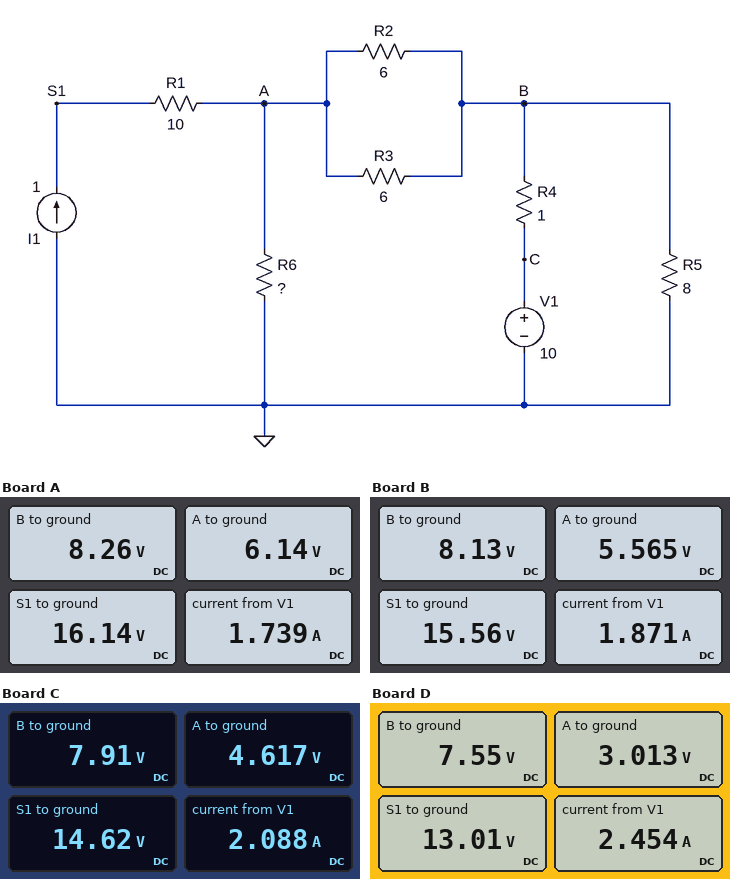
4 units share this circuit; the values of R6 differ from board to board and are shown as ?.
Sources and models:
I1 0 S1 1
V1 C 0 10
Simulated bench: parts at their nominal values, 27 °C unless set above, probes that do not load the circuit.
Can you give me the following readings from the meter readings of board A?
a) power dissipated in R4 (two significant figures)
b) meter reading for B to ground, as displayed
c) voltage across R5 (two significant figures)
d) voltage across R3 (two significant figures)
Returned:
3.0 W
8.26 V
8.3 V
2.1 V
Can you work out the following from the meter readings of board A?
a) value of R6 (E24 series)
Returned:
3.6 Ω
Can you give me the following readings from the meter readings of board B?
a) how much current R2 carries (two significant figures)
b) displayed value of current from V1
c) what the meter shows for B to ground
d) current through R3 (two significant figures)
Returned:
430 mA
1.871 A
8.13 V
430 mA
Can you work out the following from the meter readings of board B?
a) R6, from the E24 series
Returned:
3 Ω
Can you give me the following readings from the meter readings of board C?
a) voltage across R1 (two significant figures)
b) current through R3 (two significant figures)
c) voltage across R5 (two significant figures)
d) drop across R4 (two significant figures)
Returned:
10 V
550 mA
7.9 V
2.1 V
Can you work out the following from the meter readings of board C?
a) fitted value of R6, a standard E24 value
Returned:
2.2 Ω
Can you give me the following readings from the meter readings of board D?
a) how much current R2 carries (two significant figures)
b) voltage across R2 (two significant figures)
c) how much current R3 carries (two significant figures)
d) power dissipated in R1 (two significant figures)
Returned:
760 mA
4.5 V
760 mA
10 W
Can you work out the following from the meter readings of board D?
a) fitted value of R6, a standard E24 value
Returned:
1.2 Ω
